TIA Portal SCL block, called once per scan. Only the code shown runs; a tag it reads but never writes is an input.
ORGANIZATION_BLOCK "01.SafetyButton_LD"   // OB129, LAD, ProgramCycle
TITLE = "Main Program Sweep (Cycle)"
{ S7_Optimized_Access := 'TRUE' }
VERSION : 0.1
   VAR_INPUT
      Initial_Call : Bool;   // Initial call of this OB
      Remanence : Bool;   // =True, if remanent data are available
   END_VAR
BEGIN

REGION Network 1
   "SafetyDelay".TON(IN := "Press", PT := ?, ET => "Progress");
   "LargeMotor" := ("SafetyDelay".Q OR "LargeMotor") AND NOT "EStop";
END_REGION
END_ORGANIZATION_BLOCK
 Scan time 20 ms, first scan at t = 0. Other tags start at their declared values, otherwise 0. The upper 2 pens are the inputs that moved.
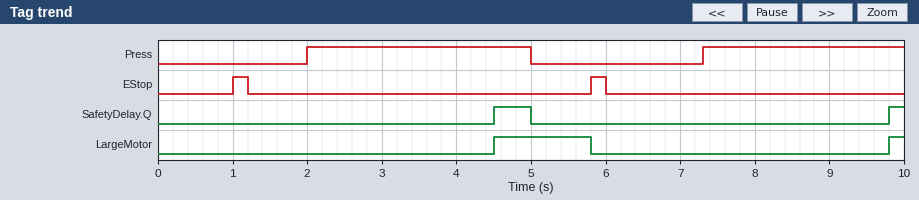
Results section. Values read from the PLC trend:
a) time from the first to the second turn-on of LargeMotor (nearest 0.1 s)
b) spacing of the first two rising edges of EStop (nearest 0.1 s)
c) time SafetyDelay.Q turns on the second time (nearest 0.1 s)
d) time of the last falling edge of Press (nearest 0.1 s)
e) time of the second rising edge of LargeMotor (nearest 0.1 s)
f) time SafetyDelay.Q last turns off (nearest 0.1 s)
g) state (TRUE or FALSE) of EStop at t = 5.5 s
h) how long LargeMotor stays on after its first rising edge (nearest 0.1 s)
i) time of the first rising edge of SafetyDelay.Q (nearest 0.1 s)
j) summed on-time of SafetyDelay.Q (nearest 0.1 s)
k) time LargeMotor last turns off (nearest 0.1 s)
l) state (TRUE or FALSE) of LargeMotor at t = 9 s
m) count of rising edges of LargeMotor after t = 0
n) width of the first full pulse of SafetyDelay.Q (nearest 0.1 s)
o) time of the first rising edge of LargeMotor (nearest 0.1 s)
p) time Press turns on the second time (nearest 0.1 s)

5.3 s
4.8 s
9.8 s
5.0 s
9.8 s
5.0 s
FALSE
1.3 s
4.5 s
0.7 s
5.8 s
FALSE
2
0.5 s
4.5 s
7.3 s
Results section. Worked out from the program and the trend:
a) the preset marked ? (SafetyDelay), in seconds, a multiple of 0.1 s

2.5 s
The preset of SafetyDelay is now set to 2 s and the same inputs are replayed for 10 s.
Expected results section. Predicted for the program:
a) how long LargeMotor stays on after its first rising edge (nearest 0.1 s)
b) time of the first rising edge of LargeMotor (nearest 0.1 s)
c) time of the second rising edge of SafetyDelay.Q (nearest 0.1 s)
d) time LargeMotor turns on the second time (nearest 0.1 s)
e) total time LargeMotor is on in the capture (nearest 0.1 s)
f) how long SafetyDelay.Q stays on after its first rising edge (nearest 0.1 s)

1.8 s
4.0 s
9.3 s
9.3 s
2.5 s
1.0 s
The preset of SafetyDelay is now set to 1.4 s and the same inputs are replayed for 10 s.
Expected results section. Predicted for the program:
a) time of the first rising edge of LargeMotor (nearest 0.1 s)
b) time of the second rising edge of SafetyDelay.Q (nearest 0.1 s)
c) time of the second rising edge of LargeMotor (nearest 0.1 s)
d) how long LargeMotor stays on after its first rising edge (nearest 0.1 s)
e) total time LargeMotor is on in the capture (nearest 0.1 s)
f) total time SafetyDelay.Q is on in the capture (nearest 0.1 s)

3.4 s
8.7 s
8.7 s
2.4 s
3.7 s
2.9 s
